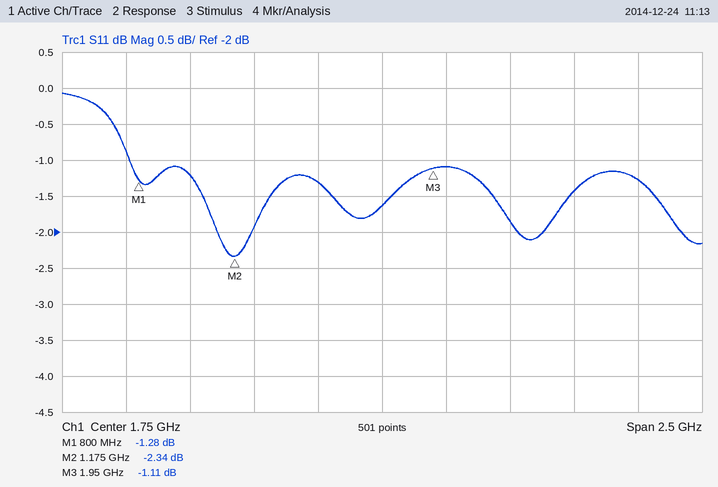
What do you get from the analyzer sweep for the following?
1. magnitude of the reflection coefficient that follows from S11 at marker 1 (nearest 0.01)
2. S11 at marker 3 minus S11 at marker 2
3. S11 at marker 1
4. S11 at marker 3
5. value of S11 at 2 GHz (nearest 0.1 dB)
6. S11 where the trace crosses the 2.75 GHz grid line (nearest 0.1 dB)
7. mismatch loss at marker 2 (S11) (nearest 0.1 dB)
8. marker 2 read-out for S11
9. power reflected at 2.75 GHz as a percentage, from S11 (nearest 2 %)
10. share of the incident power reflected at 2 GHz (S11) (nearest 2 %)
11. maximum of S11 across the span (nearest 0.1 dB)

0.86
1.23 dB
-1.28 dB
-1.11 dB
-1.1 dB
-1.3 dB
3.8 dB
-2.34 dB
74 %
78 %
-0.1 dB
